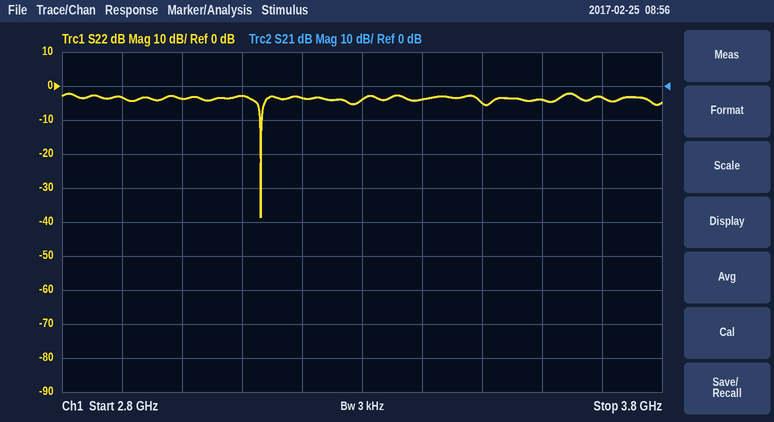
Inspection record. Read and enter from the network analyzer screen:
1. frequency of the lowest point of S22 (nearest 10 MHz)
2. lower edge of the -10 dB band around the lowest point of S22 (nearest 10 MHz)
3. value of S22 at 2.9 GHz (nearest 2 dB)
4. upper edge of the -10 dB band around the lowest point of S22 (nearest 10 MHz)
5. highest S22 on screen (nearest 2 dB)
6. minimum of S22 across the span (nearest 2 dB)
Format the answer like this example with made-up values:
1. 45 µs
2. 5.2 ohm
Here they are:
1. 3.13 GHz
2. 3.13 GHz
3. -4 dB
4. 3.13 GHz
5. -2 dB
6. -38 dB
